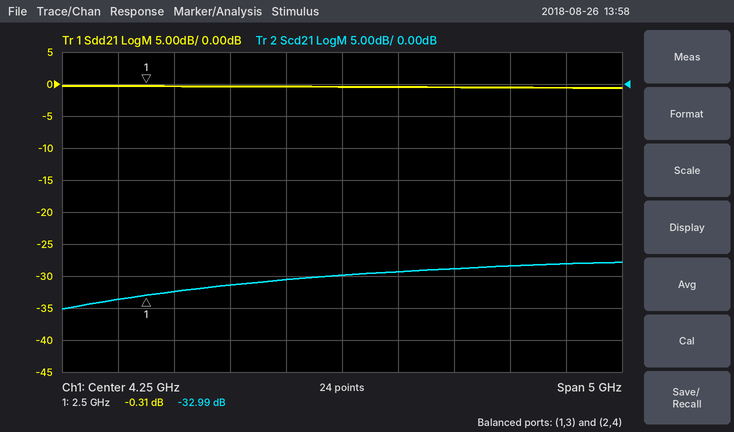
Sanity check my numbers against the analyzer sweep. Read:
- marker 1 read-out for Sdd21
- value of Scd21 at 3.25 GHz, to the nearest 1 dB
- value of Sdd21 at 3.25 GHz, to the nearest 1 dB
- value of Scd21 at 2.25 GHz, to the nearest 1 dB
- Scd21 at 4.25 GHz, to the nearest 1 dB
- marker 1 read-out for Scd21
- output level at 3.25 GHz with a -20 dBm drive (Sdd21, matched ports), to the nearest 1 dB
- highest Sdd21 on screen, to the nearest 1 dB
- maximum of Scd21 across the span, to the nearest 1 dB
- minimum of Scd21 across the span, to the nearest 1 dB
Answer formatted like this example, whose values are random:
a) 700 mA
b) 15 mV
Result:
a) -0.31 dB
b) -31 dB
c) 0 dB
d) -34 dB
e) -30 dB
f) -32.99 dB
g) -20 dBm
h) 0 dB
i) -28 dB
j) -35 dB
